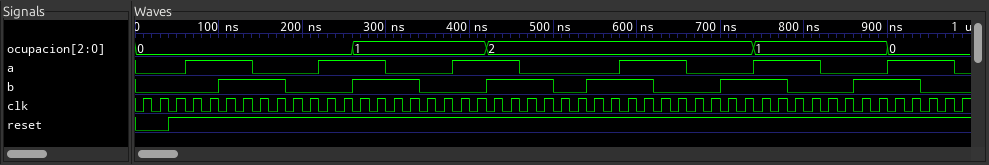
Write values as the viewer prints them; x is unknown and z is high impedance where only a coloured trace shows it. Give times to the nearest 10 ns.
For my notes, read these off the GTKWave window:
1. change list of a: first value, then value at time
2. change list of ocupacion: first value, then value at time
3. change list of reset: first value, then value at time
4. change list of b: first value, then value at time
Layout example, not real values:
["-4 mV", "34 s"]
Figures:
["0, 1 at 60 ns, 0 at 140 ns, 1 at 220 ns, 0 at 300 ns, 1 at 380 ns, 0 at 460 ns, 1 at 580 ns, 0 at 660 ns, 1 at 740 ns, 0 at 820 ns, 1 at 900 ns, 0 at 980 ns", "0, 1 at 260 ns, 2 at 420 ns, 1 at 740 ns, 0 at 900 ns", "0, 1 at 40 ns", "0, 1 at 100 ns, 0 at 180 ns, 1 at 260 ns, 0 at 340 ns, 1 at 420 ns, 0 at 500 ns, 1 at 540 ns, 0 at 620 ns, 1 at 700 ns, 0 at 780 ns, 1 at 860 ns, 0 at 940 ns"]
